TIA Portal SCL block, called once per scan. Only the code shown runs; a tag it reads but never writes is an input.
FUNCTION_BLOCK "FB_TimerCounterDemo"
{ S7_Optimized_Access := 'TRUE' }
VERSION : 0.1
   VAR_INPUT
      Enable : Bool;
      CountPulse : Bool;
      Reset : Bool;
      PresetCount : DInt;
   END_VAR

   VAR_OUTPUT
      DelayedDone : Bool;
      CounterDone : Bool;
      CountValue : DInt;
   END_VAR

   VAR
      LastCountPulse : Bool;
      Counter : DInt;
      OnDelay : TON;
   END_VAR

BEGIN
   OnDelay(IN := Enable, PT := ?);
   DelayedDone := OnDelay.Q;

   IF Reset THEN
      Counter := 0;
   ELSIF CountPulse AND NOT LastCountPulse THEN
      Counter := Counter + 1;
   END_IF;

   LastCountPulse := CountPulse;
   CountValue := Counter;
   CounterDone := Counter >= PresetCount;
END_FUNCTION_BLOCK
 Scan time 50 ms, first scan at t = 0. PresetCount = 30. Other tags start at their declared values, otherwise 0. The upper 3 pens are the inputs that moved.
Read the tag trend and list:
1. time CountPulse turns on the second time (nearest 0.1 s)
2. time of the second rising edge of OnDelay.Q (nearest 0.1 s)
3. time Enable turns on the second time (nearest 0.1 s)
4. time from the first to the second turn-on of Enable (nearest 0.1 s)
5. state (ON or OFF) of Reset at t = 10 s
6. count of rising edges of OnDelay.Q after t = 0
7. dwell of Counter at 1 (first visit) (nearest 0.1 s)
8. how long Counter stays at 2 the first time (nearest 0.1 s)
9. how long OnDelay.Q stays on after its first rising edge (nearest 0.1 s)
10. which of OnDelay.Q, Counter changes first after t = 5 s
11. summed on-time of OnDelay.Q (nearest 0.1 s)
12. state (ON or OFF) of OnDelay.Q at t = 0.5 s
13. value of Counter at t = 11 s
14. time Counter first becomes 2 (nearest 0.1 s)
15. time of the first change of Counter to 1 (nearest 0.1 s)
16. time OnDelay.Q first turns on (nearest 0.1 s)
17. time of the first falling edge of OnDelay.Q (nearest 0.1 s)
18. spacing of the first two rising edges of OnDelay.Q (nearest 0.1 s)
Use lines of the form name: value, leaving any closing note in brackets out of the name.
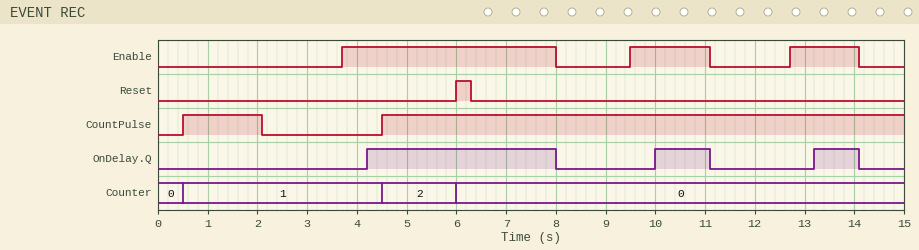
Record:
time CountPulse turns on the second time: 4.5 s
time of the second rising edge of OnDelay.Q: 10.0 s
time Enable turns on the second time: 9.5 s
time from the first to the second turn-on of Enable: 5.8 s
state (ON or OFF) of Reset at t = 10 s: OFF
count of rising edges of OnDelay.Q after t = 0: 3
dwell of Counter at 1 (first visit): 4.0 s
how long Counter stays at 2 the first time: 1.5 s
how long OnDelay.Q stays on after its first rising edge: 3.8 s
which of OnDelay.Q, Counter changes first after t = 5 s: Counter
summed on-time of OnDelay.Q: 5.8 s
state (ON or OFF) of OnDelay.Q at t = 0.5 s: OFF
value of Counter at t = 11 s: 0
time Counter first becomes 2: 4.5 s
time of the first change of Counter to 1: 0.5 s
time OnDelay.Q first turns on: 4.2 s
time of the first falling edge of OnDelay.Q: 8.0 s
spacing of the first two rising edges of OnDelay.Q: 5.8 s
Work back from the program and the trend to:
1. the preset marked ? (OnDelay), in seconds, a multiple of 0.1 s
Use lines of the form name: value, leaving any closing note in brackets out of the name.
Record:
the preset marked ? (OnDelay), in seconds, a multiple of 0.1 s: 0.5 s
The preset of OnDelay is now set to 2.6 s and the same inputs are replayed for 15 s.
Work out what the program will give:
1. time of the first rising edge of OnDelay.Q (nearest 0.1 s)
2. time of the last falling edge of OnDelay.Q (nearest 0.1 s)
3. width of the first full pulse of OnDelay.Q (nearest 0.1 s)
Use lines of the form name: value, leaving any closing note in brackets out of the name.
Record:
time of the first rising edge of OnDelay.Q: 6.3 s
time of the last falling edge of OnDelay.Q: 8.0 s
width of the first full pulse of OnDelay.Q: 1.7 s
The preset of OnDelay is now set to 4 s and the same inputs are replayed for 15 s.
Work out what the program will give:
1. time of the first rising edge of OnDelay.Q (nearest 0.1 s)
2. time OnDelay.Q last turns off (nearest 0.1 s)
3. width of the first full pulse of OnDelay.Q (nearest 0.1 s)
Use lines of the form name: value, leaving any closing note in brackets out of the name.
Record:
time of the first rising edge of OnDelay.Q: 7.7 s
time OnDelay.Q last turns off: 8.0 s
width of the first full pulse of OnDelay.Q: 0.3 s
